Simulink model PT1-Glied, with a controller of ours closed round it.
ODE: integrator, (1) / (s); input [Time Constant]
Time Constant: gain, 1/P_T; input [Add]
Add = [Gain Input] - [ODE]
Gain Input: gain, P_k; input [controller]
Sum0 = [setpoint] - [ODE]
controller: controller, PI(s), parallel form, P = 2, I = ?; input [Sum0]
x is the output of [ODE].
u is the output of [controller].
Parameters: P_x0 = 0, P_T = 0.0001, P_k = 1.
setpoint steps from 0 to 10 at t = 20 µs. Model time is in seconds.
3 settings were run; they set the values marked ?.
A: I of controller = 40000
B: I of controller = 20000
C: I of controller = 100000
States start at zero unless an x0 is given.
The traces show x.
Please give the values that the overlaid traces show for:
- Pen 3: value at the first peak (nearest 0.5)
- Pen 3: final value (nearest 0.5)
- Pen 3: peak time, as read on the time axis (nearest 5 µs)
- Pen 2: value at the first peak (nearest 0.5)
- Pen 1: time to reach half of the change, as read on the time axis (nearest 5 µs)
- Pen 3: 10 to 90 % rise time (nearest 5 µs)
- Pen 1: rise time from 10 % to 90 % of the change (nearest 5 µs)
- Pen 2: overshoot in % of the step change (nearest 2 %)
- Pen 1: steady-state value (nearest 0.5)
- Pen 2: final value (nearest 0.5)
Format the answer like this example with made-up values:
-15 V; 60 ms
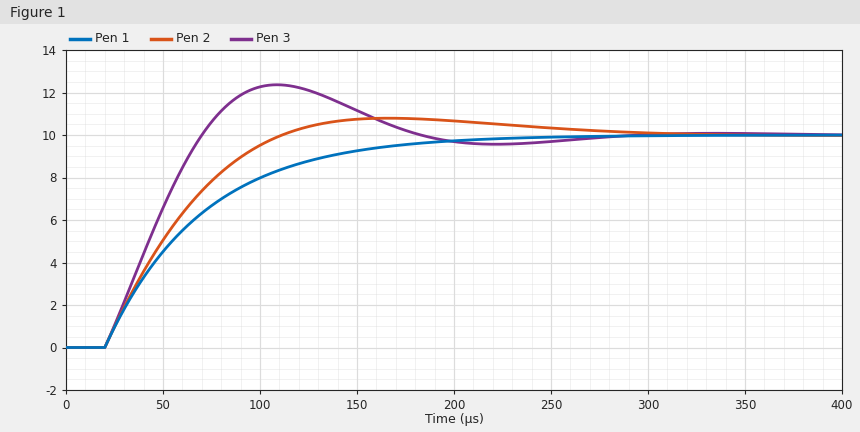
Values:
12.5; 10.0; 110 µs; 11.0; 55 µs; 40 µs; 110 µs; 8 %; 10.0; 10.0
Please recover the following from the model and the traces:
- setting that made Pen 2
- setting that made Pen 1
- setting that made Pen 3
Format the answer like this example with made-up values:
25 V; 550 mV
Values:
A; B; C
